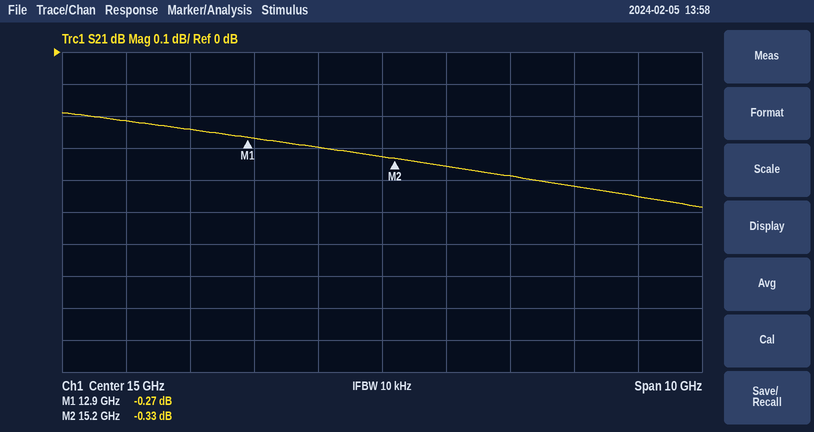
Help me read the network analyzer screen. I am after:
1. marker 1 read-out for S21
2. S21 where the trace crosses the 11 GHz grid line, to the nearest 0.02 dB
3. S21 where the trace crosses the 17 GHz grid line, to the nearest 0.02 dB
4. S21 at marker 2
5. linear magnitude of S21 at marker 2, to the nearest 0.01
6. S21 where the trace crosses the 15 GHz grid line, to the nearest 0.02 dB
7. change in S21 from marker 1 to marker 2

-0.27 dB
-0.22 dB
-0.38 dB
-0.33 dB
0.96
-0.32 dB
-0.06 dB
